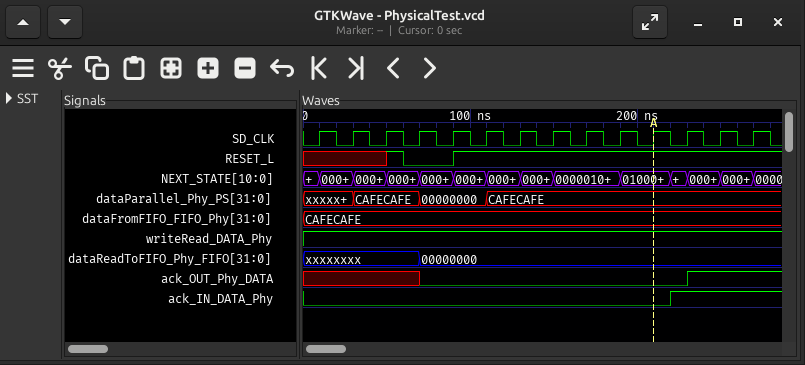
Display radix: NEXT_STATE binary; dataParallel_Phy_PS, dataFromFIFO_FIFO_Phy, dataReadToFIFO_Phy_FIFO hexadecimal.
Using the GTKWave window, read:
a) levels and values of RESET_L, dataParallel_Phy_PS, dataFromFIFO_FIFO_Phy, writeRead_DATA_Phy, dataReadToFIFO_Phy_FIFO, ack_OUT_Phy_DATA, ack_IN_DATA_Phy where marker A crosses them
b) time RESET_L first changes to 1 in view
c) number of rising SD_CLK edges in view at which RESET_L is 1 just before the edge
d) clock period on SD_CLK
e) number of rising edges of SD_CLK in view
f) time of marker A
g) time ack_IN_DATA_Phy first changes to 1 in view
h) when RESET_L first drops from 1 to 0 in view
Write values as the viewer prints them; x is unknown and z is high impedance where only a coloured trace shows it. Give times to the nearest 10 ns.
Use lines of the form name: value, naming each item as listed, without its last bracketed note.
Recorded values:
levels and values of RESET_L, dataParallel_Phy_PS, dataFromFIFO_FIFO_Phy, writeRead_DATA_Phy, dataReadToFIFO_Phy_FIFO, ack_OUT_Phy_DATA, ack_IN_DATA_Phy where marker A crosses them: RESET_L=1, dataParallel_Phy_PS=CAFECAFE, dataFromFIFO_FIFO_Phy=CAFECAFE, writeRead_DATA_Phy=1, dataReadToFIFO_Phy_FIFO=00000000, ack_OUT_Phy_DATA=0, ack_IN_DATA_Phy=0
time RESET_L first changes to 1 in view: 50 ns
number of rising SD_CLK edges in view at which RESET_L is 1 just before the edge: 9
clock period on SD_CLK: 20 ns
number of rising edges of SD_CLK in view: 14
time of marker A: 210 ns
time ack_IN_DATA_Phy first changes to 1 in view: 220 ns
when RESET_L first drops from 1 to 0 in view: 60 ns
